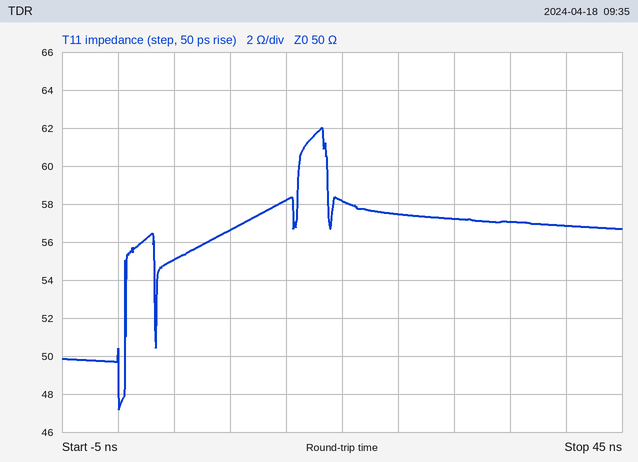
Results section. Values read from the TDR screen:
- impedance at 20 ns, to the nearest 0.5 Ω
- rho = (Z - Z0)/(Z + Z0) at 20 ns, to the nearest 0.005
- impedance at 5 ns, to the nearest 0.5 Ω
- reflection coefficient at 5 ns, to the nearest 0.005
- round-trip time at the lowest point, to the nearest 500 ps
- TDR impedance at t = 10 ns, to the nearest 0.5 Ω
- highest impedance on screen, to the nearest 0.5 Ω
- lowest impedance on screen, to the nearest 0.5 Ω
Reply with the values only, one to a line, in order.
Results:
58.0 Ω
+0.075
55.0 Ω
+0.050
0.0 ns
56.5 Ω
62.0 Ω
47.0 Ω
